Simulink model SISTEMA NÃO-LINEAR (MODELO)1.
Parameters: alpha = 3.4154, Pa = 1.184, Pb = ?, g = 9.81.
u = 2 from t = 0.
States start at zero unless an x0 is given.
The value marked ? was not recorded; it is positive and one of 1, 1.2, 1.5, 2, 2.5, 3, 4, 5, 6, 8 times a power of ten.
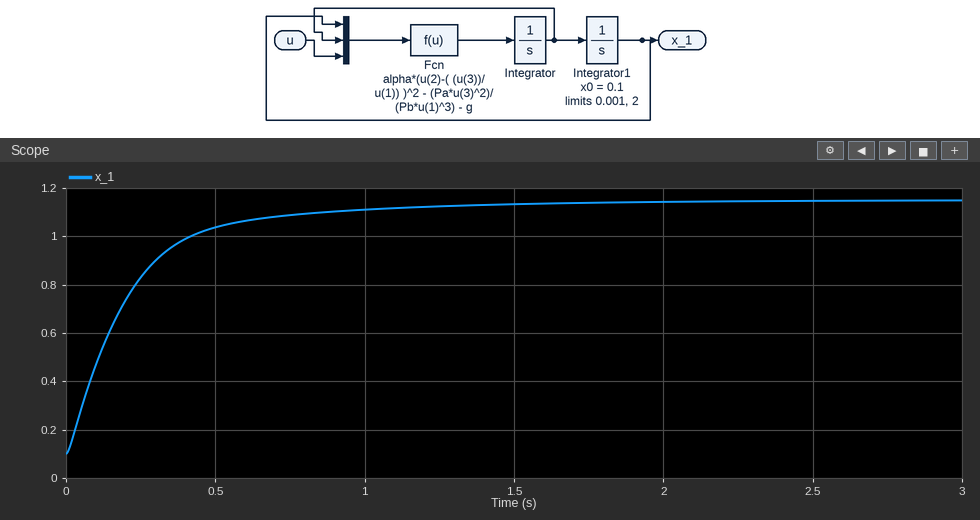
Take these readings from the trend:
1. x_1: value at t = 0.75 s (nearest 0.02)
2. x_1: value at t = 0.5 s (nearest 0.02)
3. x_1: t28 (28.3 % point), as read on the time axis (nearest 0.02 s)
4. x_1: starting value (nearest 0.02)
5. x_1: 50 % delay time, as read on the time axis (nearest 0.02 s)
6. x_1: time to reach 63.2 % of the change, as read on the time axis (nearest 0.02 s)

1.08
1.04
0.08 s
0.10
0.16 s
0.22 s
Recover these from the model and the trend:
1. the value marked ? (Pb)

6
